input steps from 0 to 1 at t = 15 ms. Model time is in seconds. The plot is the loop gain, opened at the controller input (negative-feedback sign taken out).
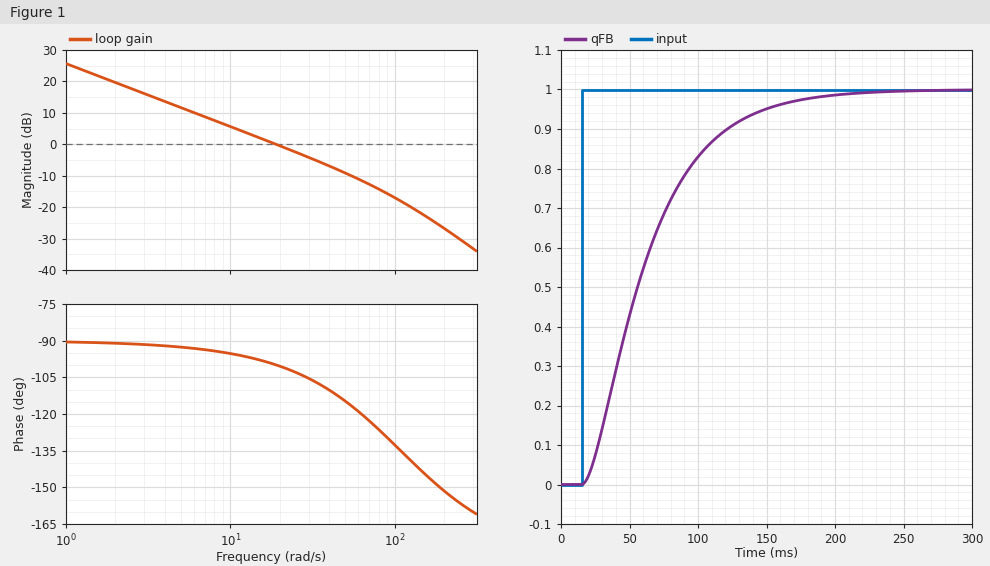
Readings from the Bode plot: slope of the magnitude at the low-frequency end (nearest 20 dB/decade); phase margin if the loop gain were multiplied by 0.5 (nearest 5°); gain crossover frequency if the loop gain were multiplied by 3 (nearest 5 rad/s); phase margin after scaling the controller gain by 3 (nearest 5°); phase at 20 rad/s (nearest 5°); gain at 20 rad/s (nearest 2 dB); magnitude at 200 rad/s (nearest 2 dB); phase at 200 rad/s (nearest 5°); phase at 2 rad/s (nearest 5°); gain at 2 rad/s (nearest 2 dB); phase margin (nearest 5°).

-20 dB/decade
85°
50 rad/s
65°
-100°
0 dB
-26 dB
-150°
-90°
20 dB
80°
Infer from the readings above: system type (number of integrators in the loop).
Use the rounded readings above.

1
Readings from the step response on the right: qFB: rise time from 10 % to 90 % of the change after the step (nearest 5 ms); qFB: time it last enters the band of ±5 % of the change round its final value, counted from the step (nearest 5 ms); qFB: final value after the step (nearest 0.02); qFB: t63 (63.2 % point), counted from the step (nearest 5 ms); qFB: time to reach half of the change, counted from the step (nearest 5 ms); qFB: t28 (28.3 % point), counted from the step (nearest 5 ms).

95 ms
135 ms
1.00
55 ms
40 ms
25 ms
